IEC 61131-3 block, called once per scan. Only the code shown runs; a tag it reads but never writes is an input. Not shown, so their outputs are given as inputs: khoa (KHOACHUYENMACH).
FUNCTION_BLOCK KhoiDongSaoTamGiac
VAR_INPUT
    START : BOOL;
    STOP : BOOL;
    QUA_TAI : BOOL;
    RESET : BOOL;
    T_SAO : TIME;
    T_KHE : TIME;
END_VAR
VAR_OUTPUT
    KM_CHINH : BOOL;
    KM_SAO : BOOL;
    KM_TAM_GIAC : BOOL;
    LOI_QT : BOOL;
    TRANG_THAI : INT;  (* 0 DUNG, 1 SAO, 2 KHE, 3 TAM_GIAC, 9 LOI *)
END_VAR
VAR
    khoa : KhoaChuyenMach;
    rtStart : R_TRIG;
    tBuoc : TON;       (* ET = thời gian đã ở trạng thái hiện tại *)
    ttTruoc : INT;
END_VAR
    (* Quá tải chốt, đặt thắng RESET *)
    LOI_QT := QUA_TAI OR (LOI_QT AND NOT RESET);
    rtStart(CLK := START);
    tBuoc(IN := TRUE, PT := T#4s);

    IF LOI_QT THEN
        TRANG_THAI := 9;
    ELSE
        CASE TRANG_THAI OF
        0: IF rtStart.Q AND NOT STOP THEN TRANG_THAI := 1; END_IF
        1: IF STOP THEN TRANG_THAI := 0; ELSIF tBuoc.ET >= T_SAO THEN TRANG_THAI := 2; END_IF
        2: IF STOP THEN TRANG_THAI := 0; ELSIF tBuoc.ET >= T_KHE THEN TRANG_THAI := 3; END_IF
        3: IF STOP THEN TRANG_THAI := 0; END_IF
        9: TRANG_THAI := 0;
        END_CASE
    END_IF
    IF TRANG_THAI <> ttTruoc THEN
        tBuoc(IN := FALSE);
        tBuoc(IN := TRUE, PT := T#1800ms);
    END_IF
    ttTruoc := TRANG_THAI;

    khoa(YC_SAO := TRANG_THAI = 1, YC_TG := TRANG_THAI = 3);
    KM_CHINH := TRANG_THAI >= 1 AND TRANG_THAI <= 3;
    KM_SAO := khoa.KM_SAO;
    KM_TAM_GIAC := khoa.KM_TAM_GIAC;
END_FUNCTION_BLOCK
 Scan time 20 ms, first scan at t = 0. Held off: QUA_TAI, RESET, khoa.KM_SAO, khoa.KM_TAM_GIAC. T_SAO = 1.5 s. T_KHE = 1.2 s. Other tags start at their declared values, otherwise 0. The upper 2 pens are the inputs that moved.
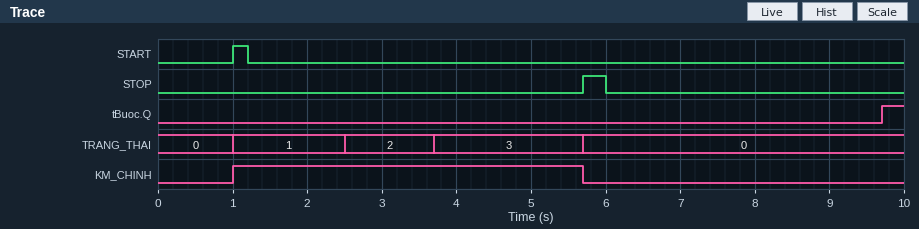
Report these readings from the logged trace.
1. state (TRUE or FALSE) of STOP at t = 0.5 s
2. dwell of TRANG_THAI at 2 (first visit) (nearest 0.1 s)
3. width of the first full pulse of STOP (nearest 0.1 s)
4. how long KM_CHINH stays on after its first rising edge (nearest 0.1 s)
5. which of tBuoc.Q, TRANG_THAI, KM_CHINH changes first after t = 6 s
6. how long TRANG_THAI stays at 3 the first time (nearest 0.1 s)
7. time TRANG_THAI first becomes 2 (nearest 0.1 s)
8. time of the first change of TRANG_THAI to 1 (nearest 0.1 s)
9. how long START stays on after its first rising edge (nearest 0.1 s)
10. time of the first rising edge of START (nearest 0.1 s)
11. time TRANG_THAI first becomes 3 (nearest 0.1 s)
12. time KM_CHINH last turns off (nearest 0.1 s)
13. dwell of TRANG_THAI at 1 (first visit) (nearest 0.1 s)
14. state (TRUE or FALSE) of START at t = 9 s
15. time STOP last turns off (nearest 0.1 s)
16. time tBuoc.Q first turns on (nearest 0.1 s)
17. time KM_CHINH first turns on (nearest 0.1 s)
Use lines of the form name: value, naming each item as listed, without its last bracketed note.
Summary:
state (TRUE or FALSE) of STOP at t = 0.5 s: FALSE
dwell of TRANG_THAI at 2 (first visit): 1.2 s
width of the first full pulse of STOP: 0.3 s
how long KM_CHINH stays on after its first rising edge: 4.7 s
which of tBuoc.Q, TRANG_THAI, KM_CHINH changes first after t = 6 s: tBuoc.Q
how long TRANG_THAI stays at 3 the first time: 2.0 s
time TRANG_THAI first becomes 2: 2.5 s
time of the first change of TRANG_THAI to 1: 1.0 s
how long START stays on after its first rising edge: 0.2 s
time of the first rising edge of START: 1.0 s
time TRANG_THAI first becomes 3: 3.7 s
time KM_CHINH last turns off: 5.7 s
dwell of TRANG_THAI at 1 (first visit): 1.5 s
state (TRUE or FALSE) of START at t = 9 s: FALSE
time STOP last turns off: 6.0 s
time tBuoc.Q first turns on: 9.7 s
time KM_CHINH first turns on: 1.0 s
